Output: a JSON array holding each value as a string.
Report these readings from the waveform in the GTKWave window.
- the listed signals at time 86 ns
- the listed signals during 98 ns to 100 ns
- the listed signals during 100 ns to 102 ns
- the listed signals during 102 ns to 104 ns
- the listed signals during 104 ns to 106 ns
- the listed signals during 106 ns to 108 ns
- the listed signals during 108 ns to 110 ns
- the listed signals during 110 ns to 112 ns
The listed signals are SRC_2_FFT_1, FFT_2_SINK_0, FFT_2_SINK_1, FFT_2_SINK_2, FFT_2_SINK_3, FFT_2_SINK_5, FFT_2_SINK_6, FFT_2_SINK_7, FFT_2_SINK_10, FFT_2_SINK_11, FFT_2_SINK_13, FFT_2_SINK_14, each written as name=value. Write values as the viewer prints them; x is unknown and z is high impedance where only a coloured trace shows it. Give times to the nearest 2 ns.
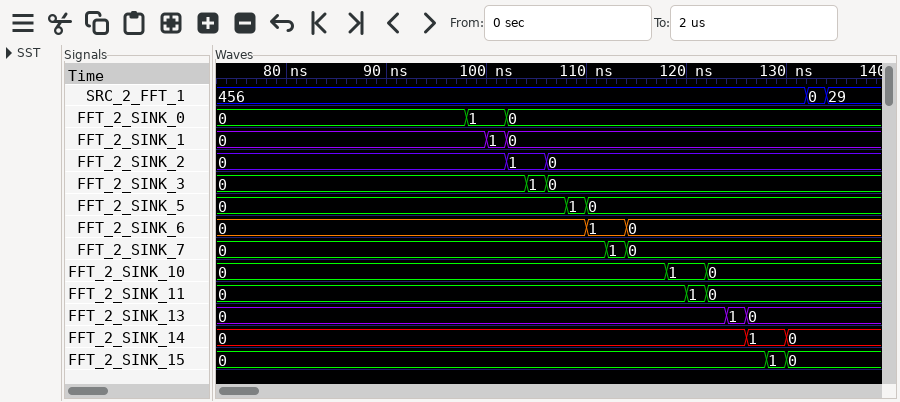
["SRC_2_FFT_1=456, FFT_2_SINK_0=0, FFT_2_SINK_1=0, FFT_2_SINK_2=0, FFT_2_SINK_3=0, FFT_2_SINK_5=0, FFT_2_SINK_6=0, FFT_2_SINK_7=0, FFT_2_SINK_10=0, FFT_2_SINK_11=0, FFT_2_SINK_13=0, FFT_2_SINK_14=0", "SRC_2_FFT_1=456, FFT_2_SINK_0=1, FFT_2_SINK_1=0, FFT_2_SINK_2=0, FFT_2_SINK_3=0, FFT_2_SINK_5=0, FFT_2_SINK_6=0, FFT_2_SINK_7=0, FFT_2_SINK_10=0, FFT_2_SINK_11=0, FFT_2_SINK_13=0, FFT_2_SINK_14=0", "SRC_2_FFT_1=456, FFT_2_SINK_0=1, FFT_2_SINK_1=1, FFT_2_SINK_2=0, FFT_2_SINK_3=0, FFT_2_SINK_5=0, FFT_2_SINK_6=0, FFT_2_SINK_7=0, FFT_2_SINK_10=0, FFT_2_SINK_11=0, FFT_2_SINK_13=0, FFT_2_SINK_14=0", "SRC_2_FFT_1=456, FFT_2_SINK_0=0, FFT_2_SINK_1=0, FFT_2_SINK_2=1, FFT_2_SINK_3=0, FFT_2_SINK_5=0, FFT_2_SINK_6=0, FFT_2_SINK_7=0, FFT_2_SINK_10=0, FFT_2_SINK_11=0, FFT_2_SINK_13=0, FFT_2_SINK_14=0", "SRC_2_FFT_1=456, FFT_2_SINK_0=0, FFT_2_SINK_1=0, FFT_2_SINK_2=1, FFT_2_SINK_3=1, FFT_2_SINK_5=0, FFT_2_SINK_6=0, FFT_2_SINK_7=0, FFT_2_SINK_10=0, FFT_2_SINK_11=0, FFT_2_SINK_13=0, FFT_2_SINK_14=0", "SRC_2_FFT_1=456, FFT_2_SINK_0=0, FFT_2_SINK_1=0, FFT_2_SINK_2=0, FFT_2_SINK_3=0, FFT_2_SINK_5=0, FFT_2_SINK_6=0, FFT_2_SINK_7=0, FFT_2_SINK_10=0, FFT_2_SINK_11=0, FFT_2_SINK_13=0, FFT_2_SINK_14=0", "SRC_2_FFT_1=456, FFT_2_SINK_0=0, FFT_2_SINK_1=0, FFT_2_SINK_2=0, FFT_2_SINK_3=0, FFT_2_SINK_5=1, FFT_2_SINK_6=0, FFT_2_SINK_7=0, FFT_2_SINK_10=0, FFT_2_SINK_11=0, FFT_2_SINK_13=0, FFT_2_SINK_14=0", "SRC_2_FFT_1=456, FFT_2_SINK_0=0, FFT_2_SINK_1=0, FFT_2_SINK_2=0, FFT_2_SINK_3=0, FFT_2_SINK_5=0, FFT_2_SINK_6=1, FFT_2_SINK_7=0, FFT_2_SINK_10=0, FFT_2_SINK_11=0, FFT_2_SINK_13=0, FFT_2_SINK_14=0"]
